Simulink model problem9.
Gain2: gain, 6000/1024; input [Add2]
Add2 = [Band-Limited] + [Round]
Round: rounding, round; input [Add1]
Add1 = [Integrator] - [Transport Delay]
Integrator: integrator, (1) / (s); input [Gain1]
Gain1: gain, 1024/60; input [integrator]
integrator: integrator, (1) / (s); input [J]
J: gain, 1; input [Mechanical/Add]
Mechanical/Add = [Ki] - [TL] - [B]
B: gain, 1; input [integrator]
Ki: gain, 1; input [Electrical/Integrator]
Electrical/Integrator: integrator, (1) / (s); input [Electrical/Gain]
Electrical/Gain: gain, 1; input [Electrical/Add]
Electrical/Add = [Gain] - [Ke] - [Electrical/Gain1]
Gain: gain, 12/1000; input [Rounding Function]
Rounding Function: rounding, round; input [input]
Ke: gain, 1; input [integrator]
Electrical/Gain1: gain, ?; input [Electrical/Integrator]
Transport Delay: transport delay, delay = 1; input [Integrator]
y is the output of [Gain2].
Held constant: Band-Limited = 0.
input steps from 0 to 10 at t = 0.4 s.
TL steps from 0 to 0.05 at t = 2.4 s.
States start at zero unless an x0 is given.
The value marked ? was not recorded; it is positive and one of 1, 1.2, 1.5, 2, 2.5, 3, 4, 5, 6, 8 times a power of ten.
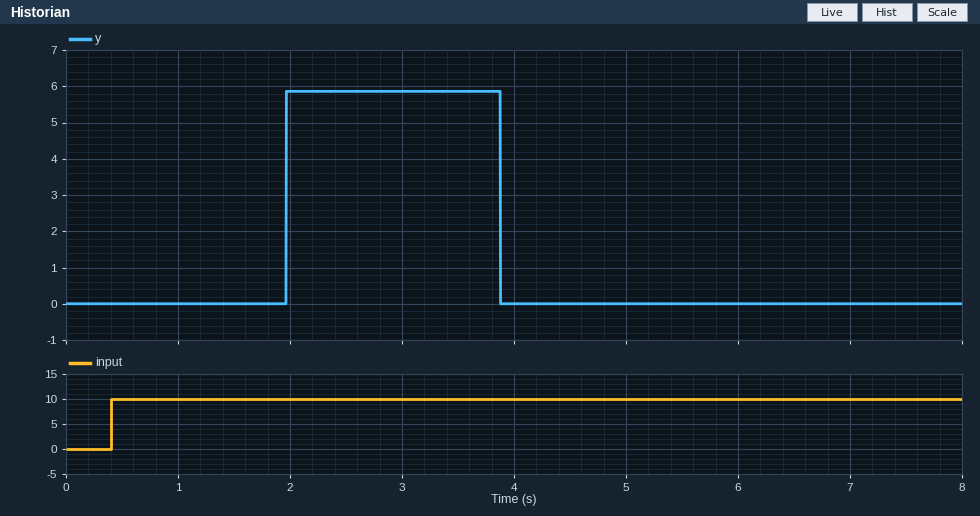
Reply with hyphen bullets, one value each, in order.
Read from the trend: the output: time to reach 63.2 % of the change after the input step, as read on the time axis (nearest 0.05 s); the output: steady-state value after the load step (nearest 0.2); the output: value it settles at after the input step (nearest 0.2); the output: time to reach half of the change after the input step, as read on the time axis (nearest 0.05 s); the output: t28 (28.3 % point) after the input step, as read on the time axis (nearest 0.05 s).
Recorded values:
- 1.95 s
- 0.0
- 5.8
- 1.95 s
- 1.95 s
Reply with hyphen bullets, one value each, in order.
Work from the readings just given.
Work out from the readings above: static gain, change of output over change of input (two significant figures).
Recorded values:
- 0.58
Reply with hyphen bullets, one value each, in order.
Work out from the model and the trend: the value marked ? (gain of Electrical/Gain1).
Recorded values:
- 1.2
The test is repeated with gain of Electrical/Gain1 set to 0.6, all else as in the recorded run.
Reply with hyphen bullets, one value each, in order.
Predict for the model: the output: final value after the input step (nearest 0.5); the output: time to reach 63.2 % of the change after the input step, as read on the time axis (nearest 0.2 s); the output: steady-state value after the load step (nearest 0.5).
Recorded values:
- 6.0
- 1.8 s
- 6.0
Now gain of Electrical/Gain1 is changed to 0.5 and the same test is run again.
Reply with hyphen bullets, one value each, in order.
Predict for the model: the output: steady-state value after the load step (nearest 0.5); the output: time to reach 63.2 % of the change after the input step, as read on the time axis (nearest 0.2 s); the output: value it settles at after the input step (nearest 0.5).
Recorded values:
- 6.0
- 1.8 s
- 6.0
